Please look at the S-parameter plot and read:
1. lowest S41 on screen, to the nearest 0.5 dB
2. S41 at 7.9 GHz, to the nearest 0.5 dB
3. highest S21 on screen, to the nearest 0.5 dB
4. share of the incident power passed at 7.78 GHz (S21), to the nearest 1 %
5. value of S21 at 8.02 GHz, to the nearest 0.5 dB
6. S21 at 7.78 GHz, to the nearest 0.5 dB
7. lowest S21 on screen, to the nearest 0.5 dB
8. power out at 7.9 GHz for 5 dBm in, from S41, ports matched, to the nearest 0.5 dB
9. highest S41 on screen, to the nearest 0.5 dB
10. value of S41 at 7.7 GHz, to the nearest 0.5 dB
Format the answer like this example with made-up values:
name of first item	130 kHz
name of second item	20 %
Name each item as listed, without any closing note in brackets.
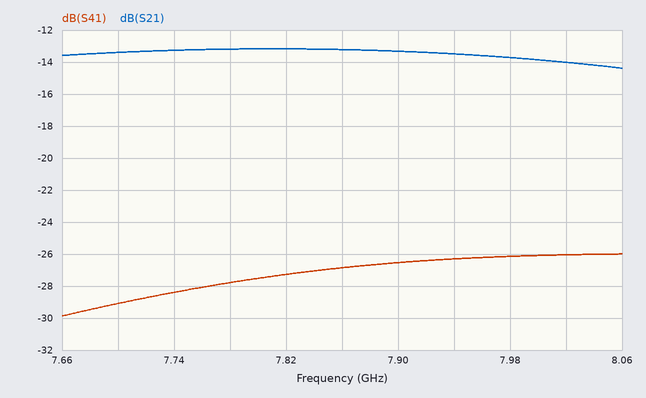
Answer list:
lowest S41 on screen, to the nearest 0.5 dB	-30.0 dB
S41 at 7.9 GHz, to the nearest 0.5 dB	-26.5 dB
highest S21 on screen, to the nearest 0.5 dB	-13.0 dB
share of the incident power passed at 7.78 GHz (S21), to the nearest 1 %	5 %
value of S21 at 8.02 GHz, to the nearest 0.5 dB	-14.0 dB
S21 at 7.78 GHz, to the nearest 0.5 dB	-13.0 dB
lowest S21 on screen, to the nearest 0.5 dB	-14.5 dB
power out at 7.9 GHz for 5 dBm in, from S41, ports matched, to the nearest 0.5 dB	-21.5 dBm
highest S41 on screen, to the nearest 0.5 dB	-26.0 dB
value of S41 at 7.7 GHz, to the nearest 0.5 dB	-29.0 dB
